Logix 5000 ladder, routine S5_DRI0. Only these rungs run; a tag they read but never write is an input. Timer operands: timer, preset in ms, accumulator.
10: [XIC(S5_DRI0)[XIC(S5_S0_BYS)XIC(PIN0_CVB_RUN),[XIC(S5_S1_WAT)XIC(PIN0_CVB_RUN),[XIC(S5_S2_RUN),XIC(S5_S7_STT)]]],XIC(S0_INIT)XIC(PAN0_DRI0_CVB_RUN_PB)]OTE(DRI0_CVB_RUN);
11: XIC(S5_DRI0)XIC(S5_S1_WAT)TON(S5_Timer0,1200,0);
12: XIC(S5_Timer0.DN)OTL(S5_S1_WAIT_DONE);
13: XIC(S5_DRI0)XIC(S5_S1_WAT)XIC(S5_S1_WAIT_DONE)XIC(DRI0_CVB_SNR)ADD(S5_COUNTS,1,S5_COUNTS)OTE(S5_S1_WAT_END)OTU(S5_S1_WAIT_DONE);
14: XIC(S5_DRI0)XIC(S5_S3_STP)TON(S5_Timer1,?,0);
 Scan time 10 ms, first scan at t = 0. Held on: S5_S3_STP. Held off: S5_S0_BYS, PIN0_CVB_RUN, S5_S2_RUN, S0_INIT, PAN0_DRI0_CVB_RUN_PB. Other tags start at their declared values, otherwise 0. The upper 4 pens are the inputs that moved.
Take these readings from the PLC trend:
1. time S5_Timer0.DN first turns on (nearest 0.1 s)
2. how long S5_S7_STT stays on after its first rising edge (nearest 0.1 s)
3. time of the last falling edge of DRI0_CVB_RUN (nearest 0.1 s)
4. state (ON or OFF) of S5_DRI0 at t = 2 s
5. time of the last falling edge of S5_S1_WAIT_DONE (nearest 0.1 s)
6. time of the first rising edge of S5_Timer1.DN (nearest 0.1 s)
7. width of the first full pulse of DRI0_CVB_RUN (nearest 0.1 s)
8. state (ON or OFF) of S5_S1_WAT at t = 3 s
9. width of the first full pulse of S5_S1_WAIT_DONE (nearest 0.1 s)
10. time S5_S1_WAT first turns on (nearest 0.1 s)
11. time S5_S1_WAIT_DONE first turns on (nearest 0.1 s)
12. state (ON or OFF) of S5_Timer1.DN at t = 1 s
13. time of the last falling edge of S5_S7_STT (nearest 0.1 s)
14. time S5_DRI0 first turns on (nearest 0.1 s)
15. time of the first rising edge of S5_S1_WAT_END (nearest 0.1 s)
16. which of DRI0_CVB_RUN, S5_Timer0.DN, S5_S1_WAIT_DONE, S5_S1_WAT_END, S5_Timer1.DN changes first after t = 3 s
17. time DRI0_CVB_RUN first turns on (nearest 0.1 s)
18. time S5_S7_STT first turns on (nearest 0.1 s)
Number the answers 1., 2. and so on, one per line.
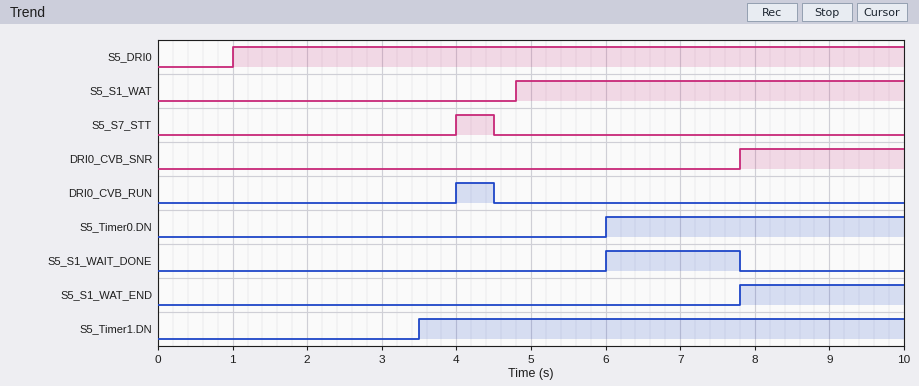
1. 6.0 s
2. 0.5 s
3. 4.5 s
4. ON
5. 7.8 s
6. 3.5 s
7. 0.5 s
8. OFF
9. 1.8 s
10. 4.8 s
11. 6.0 s
12. OFF
13. 4.5 s
14. 1.0 s
15. 7.8 s
16. S5_Timer1.DN
17. 4.0 s
18. 4.0 s
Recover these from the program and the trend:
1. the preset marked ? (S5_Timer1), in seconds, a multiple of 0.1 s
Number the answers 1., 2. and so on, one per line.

1. 2.5 s
